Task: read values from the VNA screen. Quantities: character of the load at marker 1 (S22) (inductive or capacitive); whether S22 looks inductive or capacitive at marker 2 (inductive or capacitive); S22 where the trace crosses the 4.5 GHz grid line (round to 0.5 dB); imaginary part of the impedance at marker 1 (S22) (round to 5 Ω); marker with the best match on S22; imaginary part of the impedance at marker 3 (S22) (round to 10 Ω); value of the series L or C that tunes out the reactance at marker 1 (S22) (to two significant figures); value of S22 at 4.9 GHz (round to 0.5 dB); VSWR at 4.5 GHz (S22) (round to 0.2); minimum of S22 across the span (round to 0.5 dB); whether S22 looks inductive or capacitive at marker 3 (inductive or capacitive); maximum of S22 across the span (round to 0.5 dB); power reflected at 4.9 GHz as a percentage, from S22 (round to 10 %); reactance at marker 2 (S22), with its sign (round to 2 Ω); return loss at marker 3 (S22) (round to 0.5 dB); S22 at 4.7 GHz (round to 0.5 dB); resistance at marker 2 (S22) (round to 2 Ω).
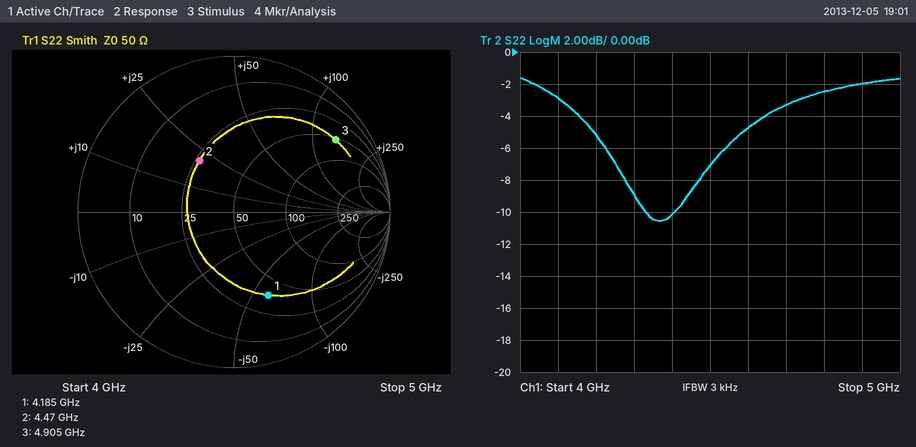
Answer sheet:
capacitive
inductive
-7.0 dB
-60 Ω
marker 2
+140 Ω
2.3 nH
-2.0 dB
2.6
-10.5 dB
inductive
-1.5 dB
60 %
+20 Ω
2.0 dB
-3.5 dB
26 Ω
